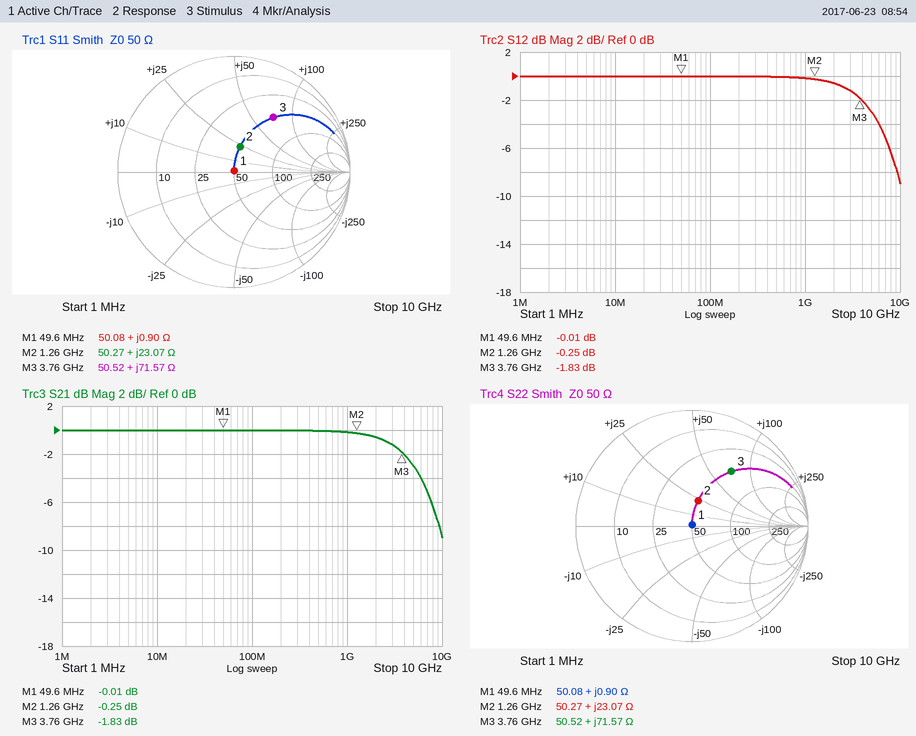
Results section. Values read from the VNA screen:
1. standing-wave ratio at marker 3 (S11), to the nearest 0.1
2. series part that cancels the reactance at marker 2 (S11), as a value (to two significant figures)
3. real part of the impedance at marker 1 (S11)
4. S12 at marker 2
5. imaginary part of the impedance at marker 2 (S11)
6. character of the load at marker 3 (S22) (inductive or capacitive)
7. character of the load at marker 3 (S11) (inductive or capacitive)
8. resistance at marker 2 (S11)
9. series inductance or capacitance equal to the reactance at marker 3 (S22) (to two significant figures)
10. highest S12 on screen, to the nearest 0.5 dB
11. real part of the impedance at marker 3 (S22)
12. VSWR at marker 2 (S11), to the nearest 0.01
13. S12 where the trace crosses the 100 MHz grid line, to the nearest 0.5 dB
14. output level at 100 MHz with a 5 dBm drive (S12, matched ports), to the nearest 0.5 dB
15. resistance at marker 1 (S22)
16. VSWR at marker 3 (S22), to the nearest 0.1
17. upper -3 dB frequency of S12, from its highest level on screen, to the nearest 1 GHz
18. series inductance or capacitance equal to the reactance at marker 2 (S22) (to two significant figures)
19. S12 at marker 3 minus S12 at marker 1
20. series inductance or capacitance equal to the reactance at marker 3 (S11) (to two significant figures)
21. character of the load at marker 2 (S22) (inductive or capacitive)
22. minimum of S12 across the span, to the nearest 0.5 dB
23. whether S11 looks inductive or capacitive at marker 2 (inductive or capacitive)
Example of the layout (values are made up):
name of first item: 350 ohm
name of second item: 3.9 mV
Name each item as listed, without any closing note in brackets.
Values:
standing-wave ratio at marker 3 (S11), to the nearest 0.1: 3.8
series part that cancels the reactance at marker 2 (S11), as a value: 5.5 pF
real part of the impedance at marker 1: 50.08 Ω
S12 at marker 2: -0.25 dB
imaginary part of the impedance at marker 2: +23.07 Ω
character of the load at marker 3 (S22): inductive
character of the load at marker 3 (S11): inductive
resistance at marker 2: 50.27 Ω
series inductance or capacitance equal to the reactance at marker 3 (S22): 3.0 nH
highest S12 on screen, to the nearest 0.5 dB: 0.0 dB
real part of the impedance at marker 3: 50.52 Ω
VSWR at marker 2 (S11), to the nearest 0.01: 1.58
S12 where the trace crosses the 100 MHz grid line, to the nearest 0.5 dB: 0.0 dB
output level at 100 MHz with a 5 dBm drive (S12, matched ports), to the nearest 0.5 dB: 5.0 dBm
resistance at marker 1: 50.08 Ω
VSWR at marker 3 (S22), to the nearest 0.1: 3.8
upper -3 dB frequency of S12, from its highest level on screen, to the nearest 1 GHz: 5 GHz
series inductance or capacitance equal to the reactance at marker 2 (S22): 2.9 nH
S12 at marker 3 minus S12 at marker 1: -1.82 dB
series inductance or capacitance equal to the reactance at marker 3 (S11): 3.0 nH
character of the load at marker 2 (S22): inductive
minimum of S12 across the span, to the nearest 0.5 dB: -9.0 dB
whether S11 looks inductive or capacitive at marker 2: inductive
